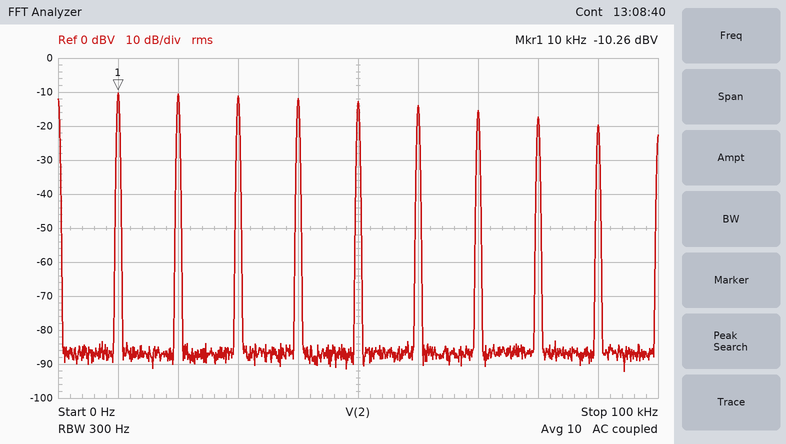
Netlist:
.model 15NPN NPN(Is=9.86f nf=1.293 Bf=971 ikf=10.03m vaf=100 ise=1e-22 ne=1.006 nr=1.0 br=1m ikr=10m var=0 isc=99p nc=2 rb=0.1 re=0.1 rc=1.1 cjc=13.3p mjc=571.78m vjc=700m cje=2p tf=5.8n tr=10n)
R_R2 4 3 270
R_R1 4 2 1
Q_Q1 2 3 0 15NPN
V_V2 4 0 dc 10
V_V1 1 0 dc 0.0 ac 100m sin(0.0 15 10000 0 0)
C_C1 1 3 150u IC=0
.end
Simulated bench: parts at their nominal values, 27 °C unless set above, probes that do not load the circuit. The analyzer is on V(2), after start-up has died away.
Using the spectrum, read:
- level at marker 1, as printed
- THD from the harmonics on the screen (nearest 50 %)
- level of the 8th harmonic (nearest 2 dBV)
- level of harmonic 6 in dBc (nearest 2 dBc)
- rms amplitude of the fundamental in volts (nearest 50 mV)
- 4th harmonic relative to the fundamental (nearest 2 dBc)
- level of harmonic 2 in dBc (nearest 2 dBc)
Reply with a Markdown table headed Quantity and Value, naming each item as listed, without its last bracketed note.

| Quantity | Value |
|---|---|
| level at marker 1, as printed | -10.26 dBV |
| THD from the harmonics on the screen | 200 % |
| level of the 8th harmonic | -18 dBV |
| level of harmonic 6 in dBc | -4 dBc |
| rms amplitude of the fundamental in volts | 300 mV |
| 4th harmonic relative to the fundamental | -2 dBc |
| level of harmonic 2 in dBc | 0 dBc |
